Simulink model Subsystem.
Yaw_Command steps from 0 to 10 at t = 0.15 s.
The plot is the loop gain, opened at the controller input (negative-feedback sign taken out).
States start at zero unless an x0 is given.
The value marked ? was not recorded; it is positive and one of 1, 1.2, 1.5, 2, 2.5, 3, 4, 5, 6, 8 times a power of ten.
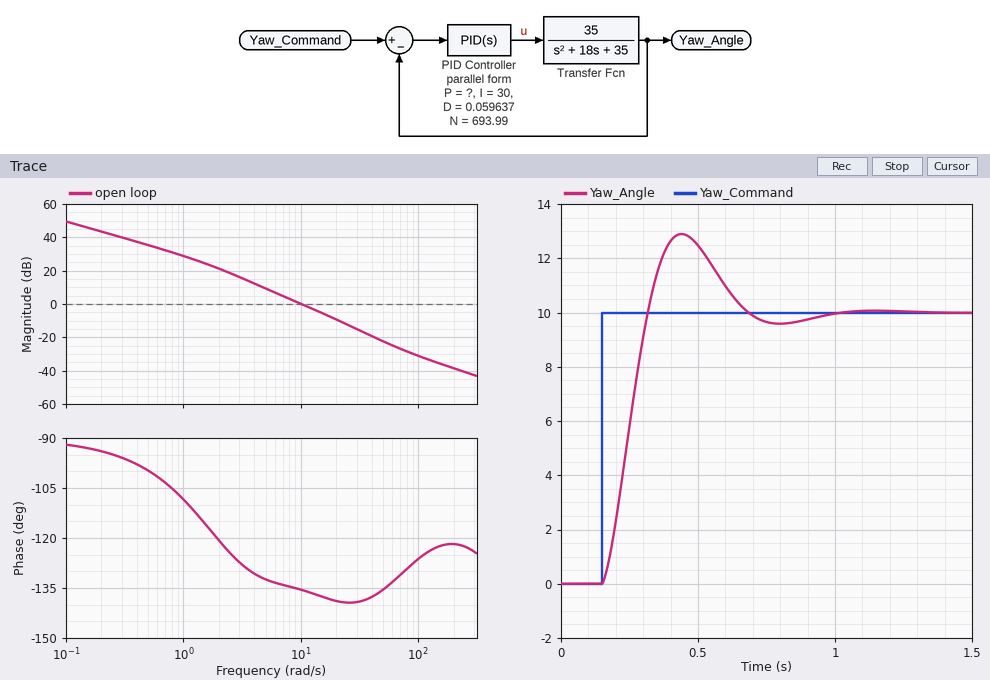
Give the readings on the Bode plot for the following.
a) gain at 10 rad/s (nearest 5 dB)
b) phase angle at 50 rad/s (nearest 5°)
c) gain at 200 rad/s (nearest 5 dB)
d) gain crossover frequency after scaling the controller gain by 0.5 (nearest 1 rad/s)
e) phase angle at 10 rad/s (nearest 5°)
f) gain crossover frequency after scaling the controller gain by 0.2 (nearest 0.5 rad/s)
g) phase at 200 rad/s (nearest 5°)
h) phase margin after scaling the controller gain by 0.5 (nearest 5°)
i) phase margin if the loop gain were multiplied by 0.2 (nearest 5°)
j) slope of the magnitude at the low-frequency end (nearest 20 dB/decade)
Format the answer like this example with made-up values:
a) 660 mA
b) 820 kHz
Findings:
a) 0 dB
b) -135°
c) -40 dB
d) 6 rad/s
e) -135°
f) 3.5 rad/s
g) -120°
h) 45°
i) 50°
j) -20 dB/decade
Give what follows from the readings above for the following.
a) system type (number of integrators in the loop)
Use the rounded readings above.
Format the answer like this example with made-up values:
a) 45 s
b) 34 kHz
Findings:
a) 1
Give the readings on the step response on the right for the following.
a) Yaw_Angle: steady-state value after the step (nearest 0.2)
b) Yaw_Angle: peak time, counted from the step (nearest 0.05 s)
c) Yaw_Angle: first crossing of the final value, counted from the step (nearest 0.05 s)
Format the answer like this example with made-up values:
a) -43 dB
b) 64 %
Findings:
a) 10.0
b) 0.30 s
c) 0.15 s
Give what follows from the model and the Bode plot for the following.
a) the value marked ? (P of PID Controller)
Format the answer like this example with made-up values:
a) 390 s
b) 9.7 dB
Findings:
a) 5
